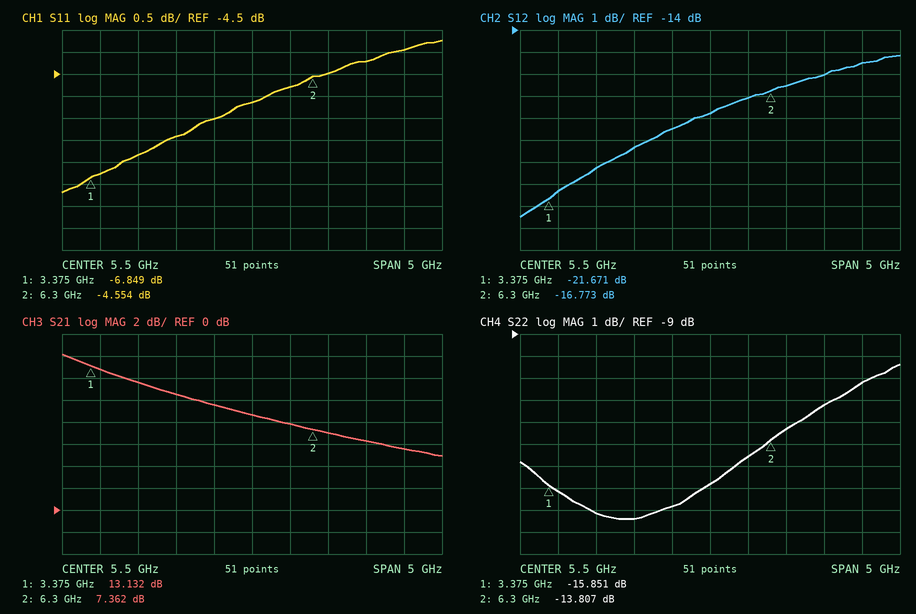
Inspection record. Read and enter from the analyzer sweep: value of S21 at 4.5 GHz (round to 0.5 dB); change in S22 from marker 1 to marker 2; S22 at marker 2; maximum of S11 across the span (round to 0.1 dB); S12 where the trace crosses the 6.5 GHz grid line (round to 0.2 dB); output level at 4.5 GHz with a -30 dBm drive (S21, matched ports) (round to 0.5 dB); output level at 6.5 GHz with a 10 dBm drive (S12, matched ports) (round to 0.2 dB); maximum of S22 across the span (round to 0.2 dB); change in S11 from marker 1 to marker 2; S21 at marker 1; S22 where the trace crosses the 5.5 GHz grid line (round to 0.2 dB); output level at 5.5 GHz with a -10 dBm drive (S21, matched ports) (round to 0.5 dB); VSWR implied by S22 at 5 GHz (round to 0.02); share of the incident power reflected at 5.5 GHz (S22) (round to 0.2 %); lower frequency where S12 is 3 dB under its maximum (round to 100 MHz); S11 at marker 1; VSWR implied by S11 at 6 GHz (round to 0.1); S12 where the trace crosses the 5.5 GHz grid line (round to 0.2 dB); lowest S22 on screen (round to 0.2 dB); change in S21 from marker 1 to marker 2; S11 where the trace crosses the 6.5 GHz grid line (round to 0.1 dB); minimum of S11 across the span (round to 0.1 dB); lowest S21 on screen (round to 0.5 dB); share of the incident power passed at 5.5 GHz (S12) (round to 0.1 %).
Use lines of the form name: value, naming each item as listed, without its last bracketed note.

value of S21 at 4.5 GHz: 10.5 dB
change in S22 from marker 1 to marker 2: 2.044 dB
S22 at marker 2: -13.807 dB
maximum of S11 across the span: -3.7 dB
S12 where the trace crosses the 6.5 GHz grid line: -16.6 dB
output level at 4.5 GHz with a -30 dBm drive (S21, matched ports): -19.5 dBm
output level at 6.5 GHz with a 10 dBm drive (S12, matched ports): -6.6 dBm
maximum of S22 across the span: -10.4 dB
change in S11 from marker 1 to marker 2: 2.295 dB
S21 at marker 1: 13.132 dB
S22 where the trace crosses the 5.5 GHz grid line: -15.8 dB
output level at 5.5 GHz with a -10 dBm drive (S21, matched ports): -1.5 dBm
VSWR implied by S22 at 5 GHz: 1.34
share of the incident power reflected at 5.5 GHz (S22): 2.6 %
lower frequency where S12 is 3 dB under its maximum: 5.2 GHz
S11 at marker 1: -6.849 dB
VSWR implied by S11 at 6 GHz: 3.7
S12 where the trace crosses the 5.5 GHz grid line: -17.8 dB
lowest S22 on screen: -17.4 dB
change in S21 from marker 1 to marker 2: -5.770 dB
S11 where the trace crosses the 6.5 GHz grid line: -4.5 dB
minimum of S11 across the span: -7.2 dB
lowest S21 on screen: 5.0 dB
share of the incident power passed at 5.5 GHz (S12): 1.7 %
